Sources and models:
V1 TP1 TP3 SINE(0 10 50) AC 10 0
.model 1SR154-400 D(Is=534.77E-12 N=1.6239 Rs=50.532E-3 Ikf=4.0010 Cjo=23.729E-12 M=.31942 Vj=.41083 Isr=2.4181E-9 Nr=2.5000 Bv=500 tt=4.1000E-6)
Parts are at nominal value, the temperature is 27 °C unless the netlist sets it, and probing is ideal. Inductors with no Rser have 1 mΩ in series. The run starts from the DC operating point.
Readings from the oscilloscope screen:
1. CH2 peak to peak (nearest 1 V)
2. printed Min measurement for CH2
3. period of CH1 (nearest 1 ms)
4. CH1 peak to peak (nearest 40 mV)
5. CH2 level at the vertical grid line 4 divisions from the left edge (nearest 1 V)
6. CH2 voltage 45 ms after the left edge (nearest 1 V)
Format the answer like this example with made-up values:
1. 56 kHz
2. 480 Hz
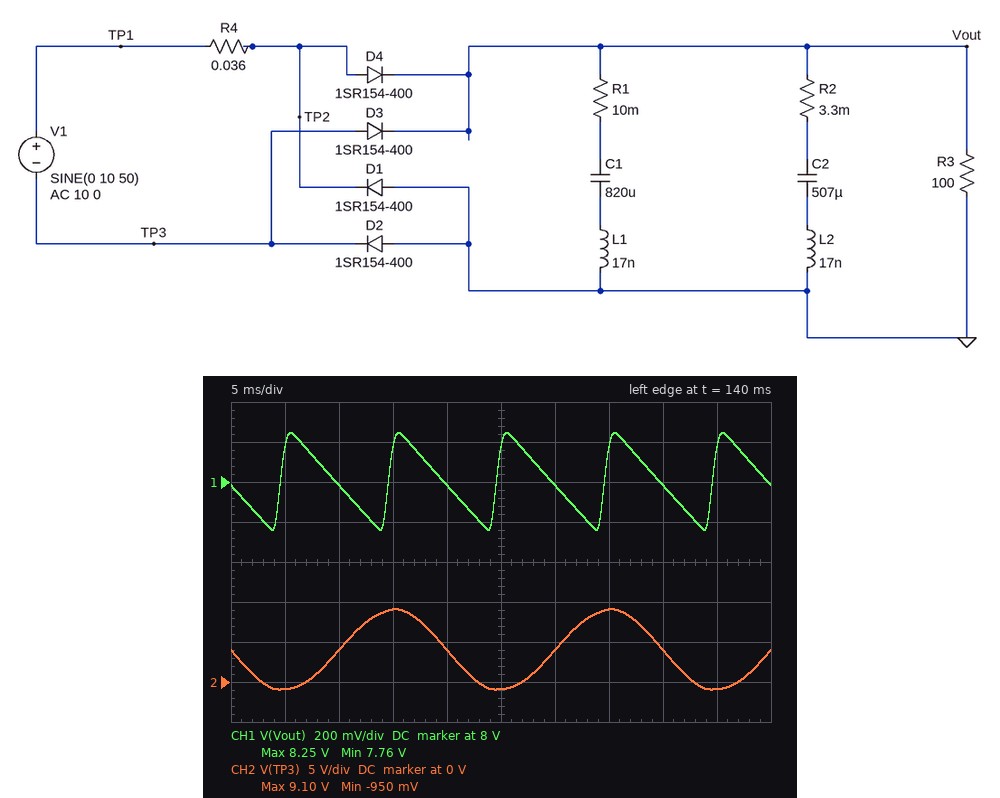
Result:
1. 10 V
2. -950 mV
3. 10 ms
4. 480 mV
5. 4 V
6. -1 V
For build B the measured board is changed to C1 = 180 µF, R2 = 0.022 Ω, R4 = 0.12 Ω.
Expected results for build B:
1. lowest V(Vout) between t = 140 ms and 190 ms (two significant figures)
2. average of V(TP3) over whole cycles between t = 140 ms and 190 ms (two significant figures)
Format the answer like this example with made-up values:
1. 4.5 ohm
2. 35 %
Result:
1. 7.4 V
2. 3.9 V
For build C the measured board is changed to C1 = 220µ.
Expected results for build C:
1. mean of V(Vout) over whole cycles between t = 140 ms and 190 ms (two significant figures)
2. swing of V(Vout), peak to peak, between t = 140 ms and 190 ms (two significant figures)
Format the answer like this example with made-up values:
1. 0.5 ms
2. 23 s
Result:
1. 7.9 V
2. 860 mV
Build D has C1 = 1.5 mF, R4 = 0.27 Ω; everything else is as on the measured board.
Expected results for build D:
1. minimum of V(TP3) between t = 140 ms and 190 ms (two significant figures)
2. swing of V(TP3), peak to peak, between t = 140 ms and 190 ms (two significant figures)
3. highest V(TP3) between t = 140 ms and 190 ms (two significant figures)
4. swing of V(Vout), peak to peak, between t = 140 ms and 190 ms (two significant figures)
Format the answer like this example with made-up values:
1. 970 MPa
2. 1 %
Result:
1. -930 mV
2. 9.9 V
3. 9.0 V
4. 310 mV
